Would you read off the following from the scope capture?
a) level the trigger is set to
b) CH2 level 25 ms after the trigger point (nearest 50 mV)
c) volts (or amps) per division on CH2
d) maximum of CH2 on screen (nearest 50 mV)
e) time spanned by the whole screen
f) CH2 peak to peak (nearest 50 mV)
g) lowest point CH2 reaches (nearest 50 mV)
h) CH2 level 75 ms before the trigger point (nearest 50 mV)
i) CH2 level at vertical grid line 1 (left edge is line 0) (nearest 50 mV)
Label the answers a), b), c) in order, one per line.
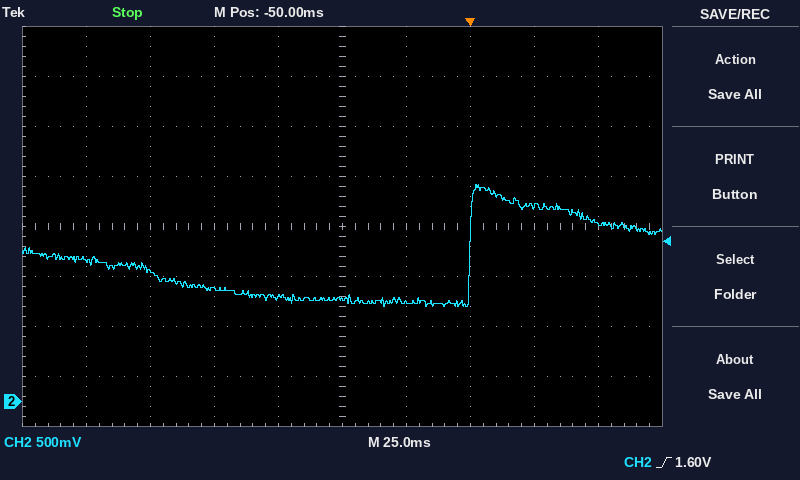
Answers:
a) 1.60 V
b) 1.95 V
c) 500 mV
d) 2.15 V
e) 250 ms
f) 1.20 V
g) 950 mV
h) 1.05 V
i) 1.40 V
